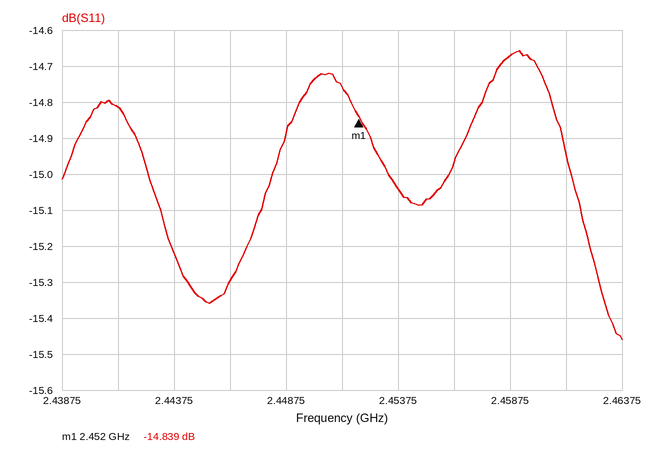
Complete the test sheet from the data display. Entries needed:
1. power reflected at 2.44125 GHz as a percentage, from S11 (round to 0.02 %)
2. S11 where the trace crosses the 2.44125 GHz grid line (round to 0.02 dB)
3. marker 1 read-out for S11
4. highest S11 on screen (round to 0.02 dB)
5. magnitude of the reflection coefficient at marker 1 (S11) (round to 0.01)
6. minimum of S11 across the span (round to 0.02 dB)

3.30 %
-14.82 dB
-14.839 dB
-14.66 dB
0.18
-15.46 dB
